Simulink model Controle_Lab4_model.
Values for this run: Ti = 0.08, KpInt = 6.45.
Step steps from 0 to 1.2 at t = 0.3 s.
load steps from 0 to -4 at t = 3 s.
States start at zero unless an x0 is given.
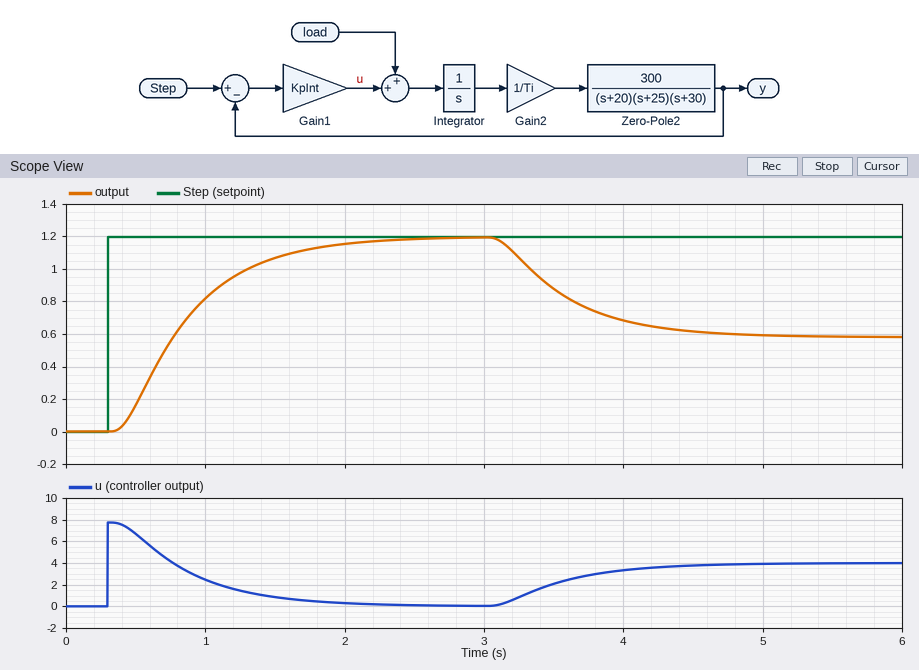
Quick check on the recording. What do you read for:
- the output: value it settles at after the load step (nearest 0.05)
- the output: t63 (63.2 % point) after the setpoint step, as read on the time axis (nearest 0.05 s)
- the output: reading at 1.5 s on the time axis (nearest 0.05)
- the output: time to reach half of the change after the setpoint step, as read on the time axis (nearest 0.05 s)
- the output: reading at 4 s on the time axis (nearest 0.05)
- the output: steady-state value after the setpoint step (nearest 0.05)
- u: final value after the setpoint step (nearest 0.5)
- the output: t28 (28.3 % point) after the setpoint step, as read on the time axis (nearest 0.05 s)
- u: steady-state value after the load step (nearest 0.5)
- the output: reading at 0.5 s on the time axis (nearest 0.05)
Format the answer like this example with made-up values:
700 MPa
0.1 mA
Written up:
0.60
0.95 s
1.05
0.80 s
0.70
1.20
0.0
0.60 s
4.0
0.15
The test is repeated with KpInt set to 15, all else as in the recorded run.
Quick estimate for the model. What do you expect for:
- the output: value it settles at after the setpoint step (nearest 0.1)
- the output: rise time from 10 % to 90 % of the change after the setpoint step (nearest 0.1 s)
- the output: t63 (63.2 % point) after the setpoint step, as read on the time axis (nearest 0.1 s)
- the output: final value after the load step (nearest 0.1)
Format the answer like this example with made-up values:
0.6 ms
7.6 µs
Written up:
1.2
0.3 s
0.6 s
0.9
